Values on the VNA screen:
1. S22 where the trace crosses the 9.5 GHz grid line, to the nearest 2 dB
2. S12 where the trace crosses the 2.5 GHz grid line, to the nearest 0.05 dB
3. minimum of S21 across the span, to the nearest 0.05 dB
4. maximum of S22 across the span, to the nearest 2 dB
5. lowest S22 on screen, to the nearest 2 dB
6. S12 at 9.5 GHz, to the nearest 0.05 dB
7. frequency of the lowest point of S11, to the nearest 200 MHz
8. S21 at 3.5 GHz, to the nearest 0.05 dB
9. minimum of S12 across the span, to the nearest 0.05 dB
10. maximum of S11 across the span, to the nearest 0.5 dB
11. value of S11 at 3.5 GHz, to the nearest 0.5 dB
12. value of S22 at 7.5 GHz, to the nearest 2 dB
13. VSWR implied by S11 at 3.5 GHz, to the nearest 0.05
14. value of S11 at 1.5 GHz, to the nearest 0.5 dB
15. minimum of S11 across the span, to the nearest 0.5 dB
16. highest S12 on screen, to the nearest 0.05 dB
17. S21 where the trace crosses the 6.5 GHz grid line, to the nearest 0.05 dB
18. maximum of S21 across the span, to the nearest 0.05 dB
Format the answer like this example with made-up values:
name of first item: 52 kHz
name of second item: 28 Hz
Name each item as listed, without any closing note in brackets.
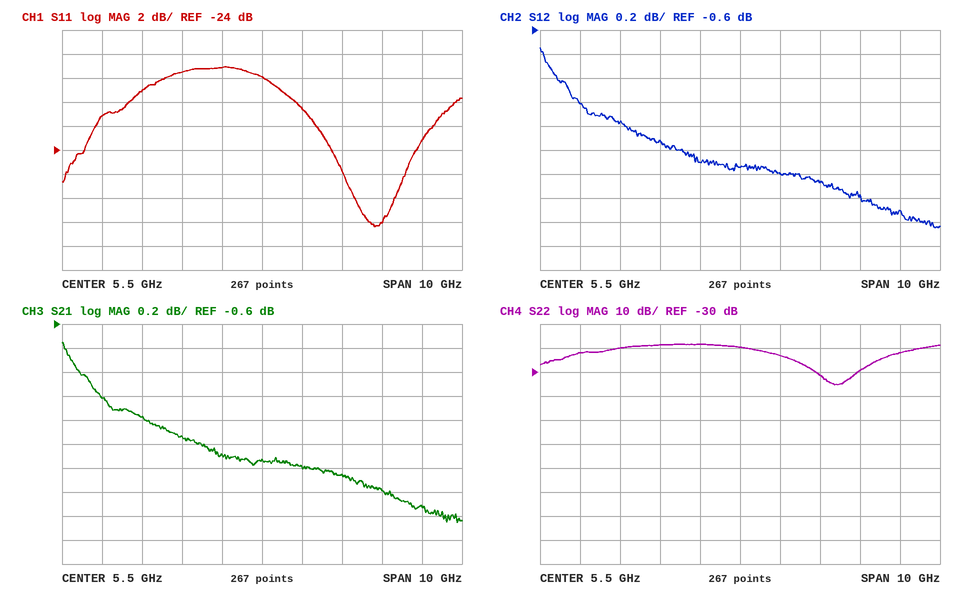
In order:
S22 where the trace crosses the 9.5 GHz grid line, to the nearest 2 dB: -22 dB
S12 where the trace crosses the 2.5 GHz grid line, to the nearest 0.05 dB: -1.35 dB
minimum of S21 across the span, to the nearest 0.05 dB: -2.25 dB
maximum of S22 across the span, to the nearest 2 dB: -18 dB
lowest S22 on screen, to the nearest 2 dB: -36 dB
S12 at 9.5 GHz, to the nearest 0.05 dB: -2.10 dB
frequency of the lowest point of S11, to the nearest 200 MHz: 8.4 GHz
S21 at 3.5 GHz, to the nearest 0.05 dB: -1.55 dB
minimum of S12 across the span, to the nearest 0.05 dB: -2.25 dB
maximum of S11 across the span, to the nearest 0.5 dB: -17.0 dB
value of S11 at 3.5 GHz, to the nearest 0.5 dB: -17.5 dB
value of S22 at 7.5 GHz, to the nearest 2 dB: -32 dB
VSWR implied by S11 at 3.5 GHz, to the nearest 0.05: 1.30
value of S11 at 1.5 GHz, to the nearest 0.5 dB: -21.0 dB
minimum of S11 across the span, to the nearest 0.5 dB: -30.5 dB
highest S12 on screen, to the nearest 0.05 dB: -0.75 dB
S21 where the trace crosses the 6.5 GHz grid line, to the nearest 0.05 dB: -1.80 dB
maximum of S21 across the span, to the nearest 0.05 dB: -0.75 dB
